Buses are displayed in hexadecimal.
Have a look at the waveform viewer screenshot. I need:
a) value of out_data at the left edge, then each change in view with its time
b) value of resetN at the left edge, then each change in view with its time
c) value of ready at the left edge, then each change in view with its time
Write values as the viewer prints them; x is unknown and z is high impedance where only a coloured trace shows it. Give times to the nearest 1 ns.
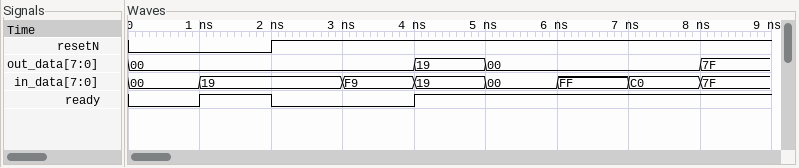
00, 19 at 4 ns, 00 at 5 ns, 7F at 8 ns
0, 1 at 2 ns
0, 1 at 1 ns, 0 at 2 ns, 1 at 4 ns
